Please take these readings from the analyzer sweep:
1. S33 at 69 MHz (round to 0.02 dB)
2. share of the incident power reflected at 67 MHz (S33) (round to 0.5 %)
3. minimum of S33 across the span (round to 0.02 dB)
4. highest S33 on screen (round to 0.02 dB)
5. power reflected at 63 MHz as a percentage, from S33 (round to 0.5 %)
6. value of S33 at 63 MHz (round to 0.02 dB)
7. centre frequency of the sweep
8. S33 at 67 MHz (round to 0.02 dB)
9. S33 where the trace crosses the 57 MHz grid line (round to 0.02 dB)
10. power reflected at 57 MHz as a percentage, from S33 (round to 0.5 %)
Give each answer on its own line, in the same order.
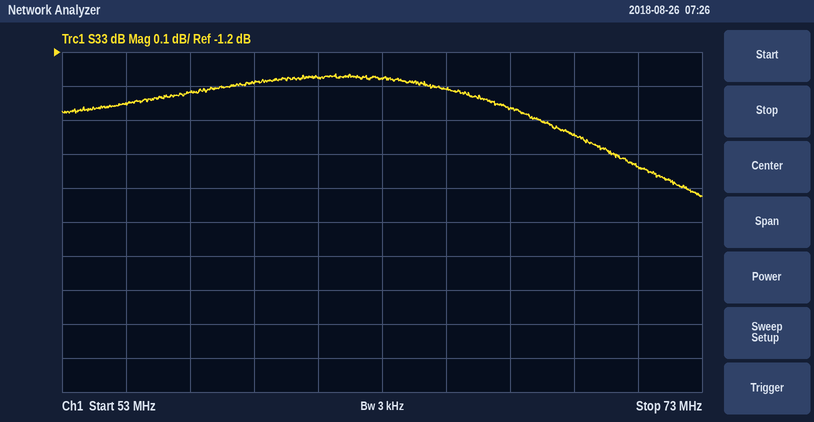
-1.44 dB
73.0 %
-1.62 dB
-1.26 dB
74.5 %
-1.28 dB
63 MHz
-1.36 dB
-1.32 dB
74.0 %
